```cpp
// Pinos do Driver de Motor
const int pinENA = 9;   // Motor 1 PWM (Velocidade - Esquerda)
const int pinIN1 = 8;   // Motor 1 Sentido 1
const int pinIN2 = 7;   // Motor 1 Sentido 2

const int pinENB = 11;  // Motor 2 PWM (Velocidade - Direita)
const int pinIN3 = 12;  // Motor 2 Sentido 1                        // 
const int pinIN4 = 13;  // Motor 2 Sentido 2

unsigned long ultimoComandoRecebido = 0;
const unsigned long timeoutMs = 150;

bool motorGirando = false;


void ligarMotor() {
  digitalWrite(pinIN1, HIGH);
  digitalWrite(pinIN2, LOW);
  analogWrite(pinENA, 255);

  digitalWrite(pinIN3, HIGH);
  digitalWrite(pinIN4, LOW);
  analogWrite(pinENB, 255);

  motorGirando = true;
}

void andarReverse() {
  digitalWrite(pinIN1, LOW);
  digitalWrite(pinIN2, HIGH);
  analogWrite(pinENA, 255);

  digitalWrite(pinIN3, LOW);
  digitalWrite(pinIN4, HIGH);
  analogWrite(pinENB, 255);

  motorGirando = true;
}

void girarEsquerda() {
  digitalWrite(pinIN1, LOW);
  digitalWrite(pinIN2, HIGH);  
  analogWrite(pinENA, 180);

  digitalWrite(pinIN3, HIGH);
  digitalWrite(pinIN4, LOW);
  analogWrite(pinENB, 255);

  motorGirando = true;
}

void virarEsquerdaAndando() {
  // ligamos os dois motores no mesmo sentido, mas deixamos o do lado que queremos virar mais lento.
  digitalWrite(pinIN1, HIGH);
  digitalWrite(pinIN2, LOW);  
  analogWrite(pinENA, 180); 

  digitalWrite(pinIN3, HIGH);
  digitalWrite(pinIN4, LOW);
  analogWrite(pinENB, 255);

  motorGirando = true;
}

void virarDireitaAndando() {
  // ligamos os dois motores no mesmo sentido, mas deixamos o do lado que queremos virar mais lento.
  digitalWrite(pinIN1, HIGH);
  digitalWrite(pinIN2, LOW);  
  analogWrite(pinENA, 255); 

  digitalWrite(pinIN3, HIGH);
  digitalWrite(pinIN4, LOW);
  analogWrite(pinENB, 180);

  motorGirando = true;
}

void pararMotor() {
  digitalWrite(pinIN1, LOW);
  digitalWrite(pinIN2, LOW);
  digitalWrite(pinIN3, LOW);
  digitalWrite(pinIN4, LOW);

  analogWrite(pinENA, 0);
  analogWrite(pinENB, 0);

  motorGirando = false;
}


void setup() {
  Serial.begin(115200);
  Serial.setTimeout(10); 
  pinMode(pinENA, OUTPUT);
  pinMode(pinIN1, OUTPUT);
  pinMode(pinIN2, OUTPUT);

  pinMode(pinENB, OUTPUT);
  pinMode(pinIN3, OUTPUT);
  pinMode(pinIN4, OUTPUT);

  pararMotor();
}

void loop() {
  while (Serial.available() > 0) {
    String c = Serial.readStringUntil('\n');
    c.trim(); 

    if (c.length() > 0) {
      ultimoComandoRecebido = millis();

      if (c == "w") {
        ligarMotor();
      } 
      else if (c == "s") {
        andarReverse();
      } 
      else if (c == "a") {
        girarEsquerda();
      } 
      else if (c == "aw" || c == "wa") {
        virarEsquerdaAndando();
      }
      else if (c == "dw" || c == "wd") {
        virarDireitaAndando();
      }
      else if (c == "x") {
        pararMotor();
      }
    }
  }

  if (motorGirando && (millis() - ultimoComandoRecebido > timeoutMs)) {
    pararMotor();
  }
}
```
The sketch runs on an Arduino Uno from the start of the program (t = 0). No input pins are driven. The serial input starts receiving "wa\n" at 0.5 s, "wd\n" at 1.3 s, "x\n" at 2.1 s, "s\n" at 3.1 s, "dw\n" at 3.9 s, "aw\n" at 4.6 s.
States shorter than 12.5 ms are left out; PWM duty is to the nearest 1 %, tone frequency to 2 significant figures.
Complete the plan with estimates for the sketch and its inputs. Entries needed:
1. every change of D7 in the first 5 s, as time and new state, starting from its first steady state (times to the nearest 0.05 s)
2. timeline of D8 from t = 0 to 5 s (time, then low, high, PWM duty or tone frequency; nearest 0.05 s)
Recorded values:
0 s low; 3.1 s high; 3.25 s low
0 s low; 0.5 s high; 0.65 s low; 1.3 s high; 1.45 s low; 3.9 s high; 4.05 s low; 4.6 s high; 4.75 s low
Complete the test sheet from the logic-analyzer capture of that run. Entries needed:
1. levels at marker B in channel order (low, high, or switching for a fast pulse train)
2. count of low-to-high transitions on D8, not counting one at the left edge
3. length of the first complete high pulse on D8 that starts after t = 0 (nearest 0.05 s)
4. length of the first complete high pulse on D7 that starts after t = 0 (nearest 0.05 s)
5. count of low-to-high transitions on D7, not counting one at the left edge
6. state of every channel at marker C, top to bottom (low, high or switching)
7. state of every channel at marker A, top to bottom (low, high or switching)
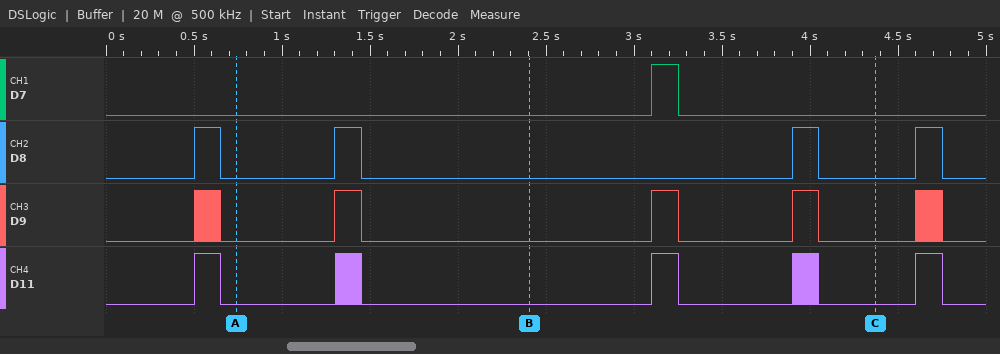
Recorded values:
D7 low, D8 low, D9 low, D11 low
4
0.15 s
0.15 s
1
D7 low, D8 low, D9 low, D11 low
D7 low, D8 low, D9 low, D11 low
